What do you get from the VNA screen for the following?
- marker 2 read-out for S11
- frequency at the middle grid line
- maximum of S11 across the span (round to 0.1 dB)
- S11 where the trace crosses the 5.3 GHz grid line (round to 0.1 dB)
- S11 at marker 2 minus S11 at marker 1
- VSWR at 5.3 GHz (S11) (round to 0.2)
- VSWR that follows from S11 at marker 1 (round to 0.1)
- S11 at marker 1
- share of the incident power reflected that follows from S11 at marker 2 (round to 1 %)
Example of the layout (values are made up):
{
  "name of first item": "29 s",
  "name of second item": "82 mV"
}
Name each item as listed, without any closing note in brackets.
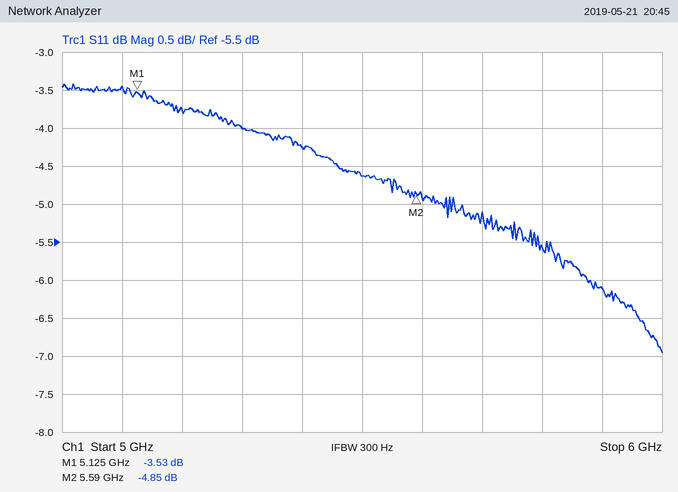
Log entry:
{
  "marker 2 read-out for S11": "-4.85 dB",
  "frequency at the middle grid line": "5.5 GHz",
  "maximum of S11 across the span": "-3.4 dB",
  "S11 where the trace crosses the 5.3 GHz grid line": "-4.0 dB",
  "S11 at marker 2 minus S11 at marker 1": "-1.32 dB",
  "VSWR at 5.3 GHz (S11)": "4.4",
  "VSWR that follows from S11 at marker 1": "5.0",
  "S11 at marker 1": "-3.53 dB",
  "share of the incident power reflected that follows from S11 at marker 2": "33 %"
}
